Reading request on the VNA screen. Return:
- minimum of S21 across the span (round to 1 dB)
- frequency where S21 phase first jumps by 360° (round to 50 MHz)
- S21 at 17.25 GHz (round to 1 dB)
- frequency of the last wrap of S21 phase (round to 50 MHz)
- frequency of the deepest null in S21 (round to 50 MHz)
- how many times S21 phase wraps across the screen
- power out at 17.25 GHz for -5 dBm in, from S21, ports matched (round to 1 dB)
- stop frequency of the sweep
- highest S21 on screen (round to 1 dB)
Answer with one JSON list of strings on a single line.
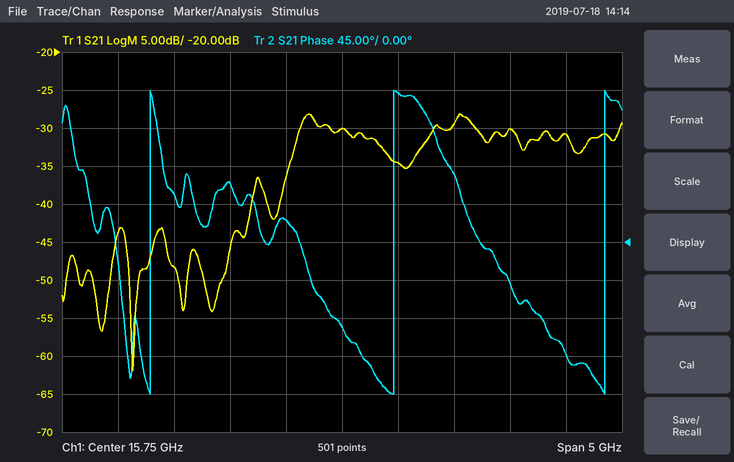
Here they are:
["-62 dB", "14.05 GHz", "-30 dB", "18.10 GHz", "13.90 GHz", "3", "-35 dBm", "18.25 GHz", "-28 dB"]
